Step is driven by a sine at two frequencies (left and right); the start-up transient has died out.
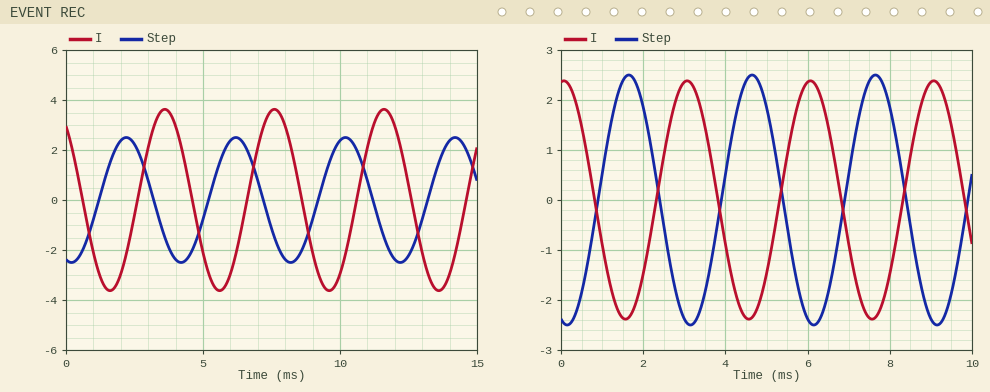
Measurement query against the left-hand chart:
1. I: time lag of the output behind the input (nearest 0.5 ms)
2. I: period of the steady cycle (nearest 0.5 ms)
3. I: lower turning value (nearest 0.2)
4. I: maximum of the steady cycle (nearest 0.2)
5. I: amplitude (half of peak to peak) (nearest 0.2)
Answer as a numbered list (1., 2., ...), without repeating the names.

1. 1.5 ms
2. 4.0 ms
3. -3.6
4. 3.6
5. 3.6
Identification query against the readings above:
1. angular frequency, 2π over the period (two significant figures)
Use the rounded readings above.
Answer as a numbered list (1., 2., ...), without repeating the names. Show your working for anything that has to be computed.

1. 2π / 4 = 1.6 rad/ms
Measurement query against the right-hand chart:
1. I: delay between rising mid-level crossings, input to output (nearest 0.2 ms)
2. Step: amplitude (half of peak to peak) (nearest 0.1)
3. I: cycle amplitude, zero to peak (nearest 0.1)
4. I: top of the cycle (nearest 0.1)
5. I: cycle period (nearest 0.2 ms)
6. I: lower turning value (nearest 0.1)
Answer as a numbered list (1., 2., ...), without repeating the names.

1. 1.4 ms
2. 2.5
3. 2.4
4. 2.4
5. 3.0 ms
6. -2.4
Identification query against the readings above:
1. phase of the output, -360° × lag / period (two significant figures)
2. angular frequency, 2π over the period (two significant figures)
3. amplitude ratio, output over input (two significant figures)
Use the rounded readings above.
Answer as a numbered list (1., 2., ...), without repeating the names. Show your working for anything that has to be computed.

1. -360 × 1.4 / 3 = -170°
2. 2π / 3 = 2.1 rad/ms
3. 2.4 / 2.5 = 0.96
